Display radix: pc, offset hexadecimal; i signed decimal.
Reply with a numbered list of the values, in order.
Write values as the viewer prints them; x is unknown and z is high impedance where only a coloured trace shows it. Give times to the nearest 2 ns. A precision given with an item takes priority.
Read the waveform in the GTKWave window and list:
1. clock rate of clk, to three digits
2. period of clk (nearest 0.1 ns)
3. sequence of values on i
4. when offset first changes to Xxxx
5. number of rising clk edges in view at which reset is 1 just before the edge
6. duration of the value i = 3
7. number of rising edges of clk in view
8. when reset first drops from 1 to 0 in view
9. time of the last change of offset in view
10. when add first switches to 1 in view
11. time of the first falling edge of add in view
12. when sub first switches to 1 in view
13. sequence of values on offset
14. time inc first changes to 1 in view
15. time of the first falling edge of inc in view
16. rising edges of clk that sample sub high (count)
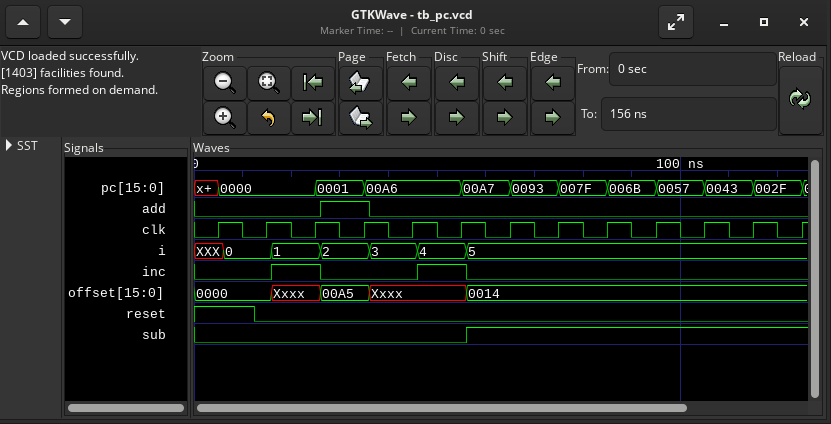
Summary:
1. 100 MHz
2. 10 ns
3. XXX, 0, 1, 2, 3, 4, 5
4. 16 ns
5. 1
6. 10 ns
7. 13
8. 12 ns
9. 56 ns
10. 26 ns
11. 36 ns
12. 56 ns
13. 0000, Xxxx, 00A5, Xxxx, 0014
14. 16 ns
15. 26 ns
16. 7
